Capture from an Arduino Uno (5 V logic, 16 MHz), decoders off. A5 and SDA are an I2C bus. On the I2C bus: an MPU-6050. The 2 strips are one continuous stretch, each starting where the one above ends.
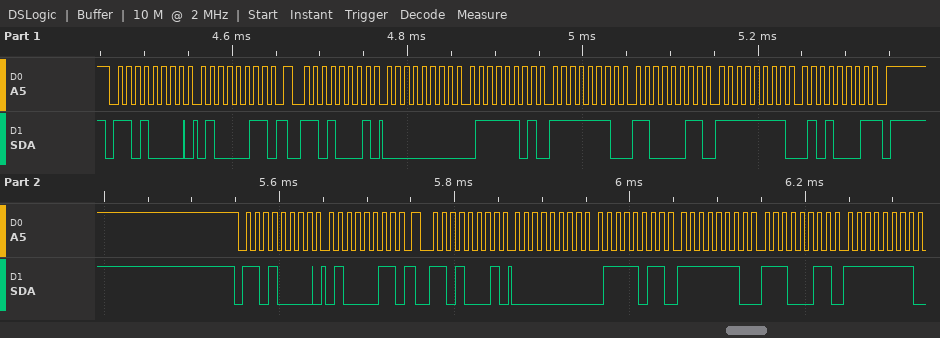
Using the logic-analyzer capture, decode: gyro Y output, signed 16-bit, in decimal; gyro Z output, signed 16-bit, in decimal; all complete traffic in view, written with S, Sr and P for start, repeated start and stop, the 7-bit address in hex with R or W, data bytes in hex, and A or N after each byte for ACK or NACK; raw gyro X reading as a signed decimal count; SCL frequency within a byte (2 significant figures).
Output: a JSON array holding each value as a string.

["-317", "-175", "S 68W A 43 A Sr 68R A 00 A 7D A FE A C3 A FF A 51 N P S 68W A 43 A Sr 68R A 00 A 7B A FE A E3 A FF A", "125", "100 kHz"]
